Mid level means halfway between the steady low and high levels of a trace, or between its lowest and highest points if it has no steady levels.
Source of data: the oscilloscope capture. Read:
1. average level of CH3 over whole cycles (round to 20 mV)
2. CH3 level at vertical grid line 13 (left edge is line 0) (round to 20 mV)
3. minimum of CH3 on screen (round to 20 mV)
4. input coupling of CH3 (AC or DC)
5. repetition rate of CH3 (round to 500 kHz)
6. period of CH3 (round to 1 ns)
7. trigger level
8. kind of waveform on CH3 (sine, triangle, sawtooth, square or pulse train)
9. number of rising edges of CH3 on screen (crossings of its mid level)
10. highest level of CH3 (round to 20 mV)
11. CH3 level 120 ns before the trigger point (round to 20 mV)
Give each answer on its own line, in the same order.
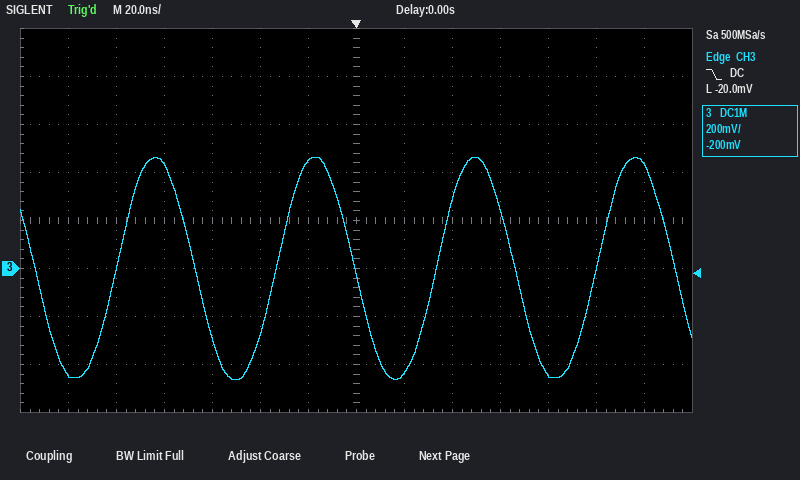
0 mV
440 mV
-460 mV
DC
15.0 MHz
67 ns
-20.0 mV
sine
4
460 mV
-440 mV
